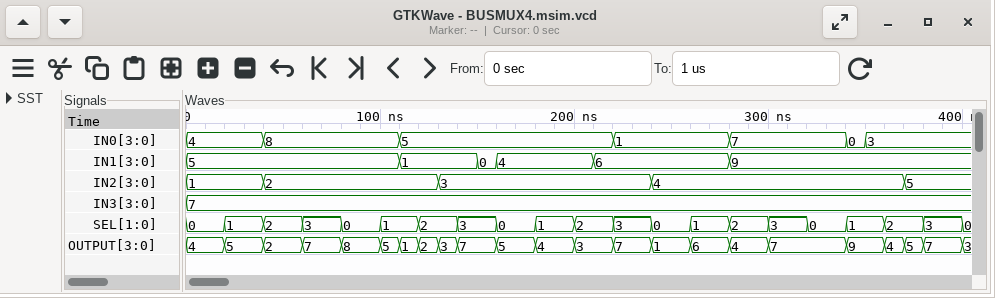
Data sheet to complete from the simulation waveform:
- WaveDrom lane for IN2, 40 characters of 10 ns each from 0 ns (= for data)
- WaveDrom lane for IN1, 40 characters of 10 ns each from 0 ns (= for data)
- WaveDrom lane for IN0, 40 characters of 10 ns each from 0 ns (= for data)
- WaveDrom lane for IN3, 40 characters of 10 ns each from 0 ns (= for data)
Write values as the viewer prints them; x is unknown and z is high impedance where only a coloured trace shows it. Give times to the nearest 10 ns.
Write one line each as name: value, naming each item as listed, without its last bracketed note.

WaveDrom lane for IN2, 40 characters of 10 ns each from 0 ns: {name: 'IN2', wave: '=...=........=..........=............=..', data: '1 2 3 4 5'}
WaveDrom lane for IN1, 40 characters of 10 ns each from 0 ns: {name: 'IN1', wave: '=..........=...==....=......=...........', data: '5 1 0 4 6 9'}
WaveDrom lane for IN0, 40 characters of 10 ns each from 0 ns: {name: 'IN0', wave: '=...=......=..........=.....=.....==....', data: '4 8 5 1 7 0 3'}
WaveDrom lane for IN3, 40 characters of 10 ns each from 0 ns: {name: 'IN3', wave: '=.......................................', data: '7'}
